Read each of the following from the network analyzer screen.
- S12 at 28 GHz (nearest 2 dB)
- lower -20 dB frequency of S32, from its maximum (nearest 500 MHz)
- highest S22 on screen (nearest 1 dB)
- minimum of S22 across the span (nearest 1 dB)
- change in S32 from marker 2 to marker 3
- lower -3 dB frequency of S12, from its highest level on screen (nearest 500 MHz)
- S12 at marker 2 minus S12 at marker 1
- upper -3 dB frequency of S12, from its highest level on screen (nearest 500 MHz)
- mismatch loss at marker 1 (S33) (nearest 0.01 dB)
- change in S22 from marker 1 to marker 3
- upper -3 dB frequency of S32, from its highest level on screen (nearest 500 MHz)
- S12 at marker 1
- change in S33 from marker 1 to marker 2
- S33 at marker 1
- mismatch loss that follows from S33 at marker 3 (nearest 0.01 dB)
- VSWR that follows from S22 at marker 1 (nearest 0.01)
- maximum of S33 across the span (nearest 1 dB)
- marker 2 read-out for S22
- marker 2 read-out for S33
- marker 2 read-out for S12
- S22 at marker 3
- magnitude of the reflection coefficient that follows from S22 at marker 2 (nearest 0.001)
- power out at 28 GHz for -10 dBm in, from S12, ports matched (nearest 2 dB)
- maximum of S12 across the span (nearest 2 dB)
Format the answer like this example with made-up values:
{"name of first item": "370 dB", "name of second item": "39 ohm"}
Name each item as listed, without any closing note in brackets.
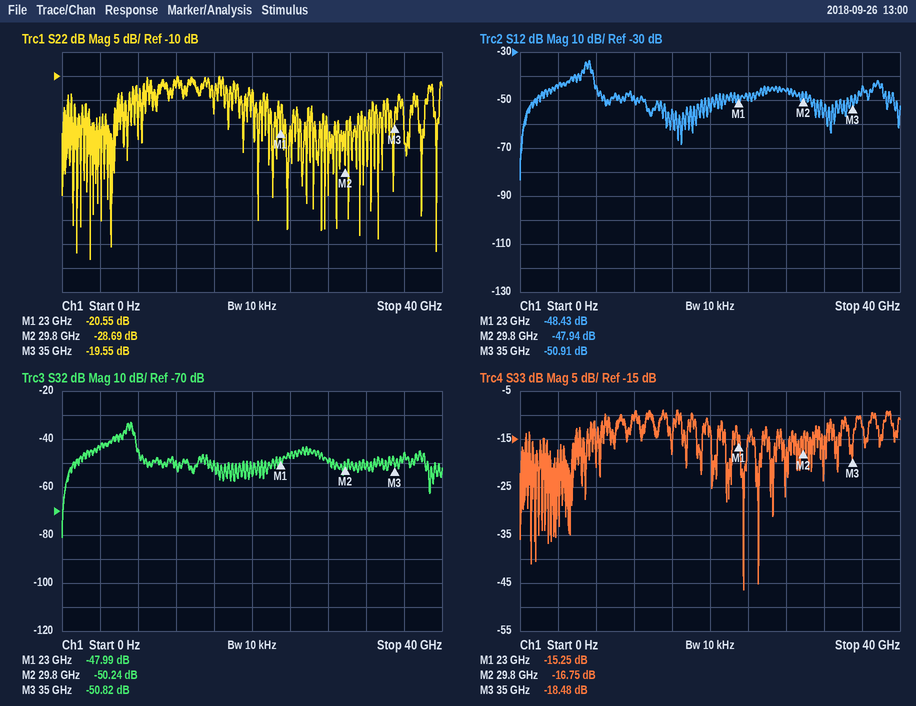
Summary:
{"S12 at 28 GHz": "-46 dB", "lower -20 dB frequency of S32, from its maximum": "1.0 GHz", "highest S22 on screen": "-10 dB", "minimum of S22 across the span": "-48 dB", "change in S32 from marker 2 to marker 3": "-0.58 dB", "lower -3 dB frequency of S12, from its highest level on screen": "7.0 GHz", "S12 at marker 2 minus S12 at marker 1": "0.49 dB", "upper -3 dB frequency of S12, from its highest level on screen": "7.5 GHz", "mismatch loss at marker 1 (S33)": "0.13 dB", "change in S22 from marker 1 to marker 3": "1.00 dB", "upper -3 dB frequency of S32, from its highest level on screen": "7.5 GHz", "S12 at marker 1": "-48.43 dB", "change in S33 from marker 1 to marker 2": "-1.50 dB", "S33 at marker 1": "-15.25 dB", "mismatch loss that follows from S33 at marker 3": "0.06 dB", "VSWR that follows from S22 at marker 1": "1.21", "maximum of S33 across the span": "-9 dB", "marker 2 read-out for S22": "-28.69 dB", "marker 2 read-out for S33": "-16.75 dB", "marker 2 read-out for S12": "-47.94 dB", "S22 at marker 3": "-19.55 dB", "magnitude of the reflection coefficient that follows from S22 at marker 2": "0.037", "power out at 28 GHz for -10 dBm in, from S12, ports matched": "-56 dBm", "maximum of S12 across the span": "-34 dB"}
